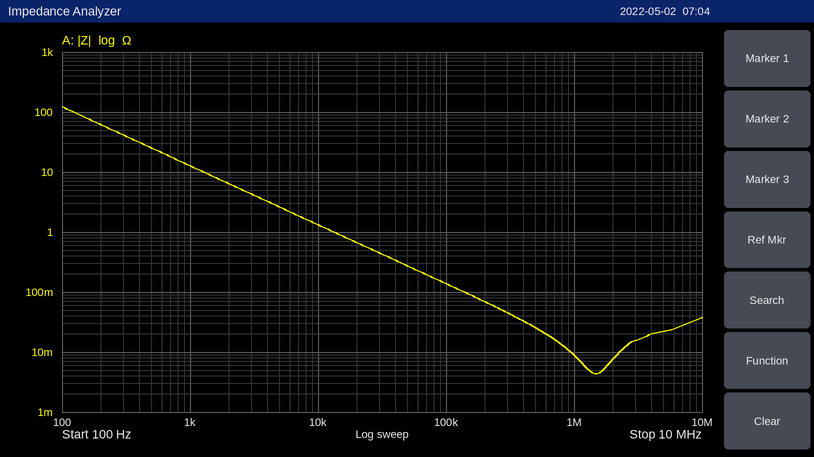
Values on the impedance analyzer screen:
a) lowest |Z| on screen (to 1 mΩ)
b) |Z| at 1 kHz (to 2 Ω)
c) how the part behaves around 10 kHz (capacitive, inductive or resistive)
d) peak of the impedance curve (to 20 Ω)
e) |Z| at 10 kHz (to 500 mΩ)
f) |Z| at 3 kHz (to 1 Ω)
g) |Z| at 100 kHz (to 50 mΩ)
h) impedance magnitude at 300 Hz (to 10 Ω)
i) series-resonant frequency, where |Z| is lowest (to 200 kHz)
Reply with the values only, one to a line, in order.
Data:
4 mΩ
12 Ω
capacitive
120 Ω
1.5 Ω
4 Ω
150 mΩ
40 Ω
1.4 MHz
